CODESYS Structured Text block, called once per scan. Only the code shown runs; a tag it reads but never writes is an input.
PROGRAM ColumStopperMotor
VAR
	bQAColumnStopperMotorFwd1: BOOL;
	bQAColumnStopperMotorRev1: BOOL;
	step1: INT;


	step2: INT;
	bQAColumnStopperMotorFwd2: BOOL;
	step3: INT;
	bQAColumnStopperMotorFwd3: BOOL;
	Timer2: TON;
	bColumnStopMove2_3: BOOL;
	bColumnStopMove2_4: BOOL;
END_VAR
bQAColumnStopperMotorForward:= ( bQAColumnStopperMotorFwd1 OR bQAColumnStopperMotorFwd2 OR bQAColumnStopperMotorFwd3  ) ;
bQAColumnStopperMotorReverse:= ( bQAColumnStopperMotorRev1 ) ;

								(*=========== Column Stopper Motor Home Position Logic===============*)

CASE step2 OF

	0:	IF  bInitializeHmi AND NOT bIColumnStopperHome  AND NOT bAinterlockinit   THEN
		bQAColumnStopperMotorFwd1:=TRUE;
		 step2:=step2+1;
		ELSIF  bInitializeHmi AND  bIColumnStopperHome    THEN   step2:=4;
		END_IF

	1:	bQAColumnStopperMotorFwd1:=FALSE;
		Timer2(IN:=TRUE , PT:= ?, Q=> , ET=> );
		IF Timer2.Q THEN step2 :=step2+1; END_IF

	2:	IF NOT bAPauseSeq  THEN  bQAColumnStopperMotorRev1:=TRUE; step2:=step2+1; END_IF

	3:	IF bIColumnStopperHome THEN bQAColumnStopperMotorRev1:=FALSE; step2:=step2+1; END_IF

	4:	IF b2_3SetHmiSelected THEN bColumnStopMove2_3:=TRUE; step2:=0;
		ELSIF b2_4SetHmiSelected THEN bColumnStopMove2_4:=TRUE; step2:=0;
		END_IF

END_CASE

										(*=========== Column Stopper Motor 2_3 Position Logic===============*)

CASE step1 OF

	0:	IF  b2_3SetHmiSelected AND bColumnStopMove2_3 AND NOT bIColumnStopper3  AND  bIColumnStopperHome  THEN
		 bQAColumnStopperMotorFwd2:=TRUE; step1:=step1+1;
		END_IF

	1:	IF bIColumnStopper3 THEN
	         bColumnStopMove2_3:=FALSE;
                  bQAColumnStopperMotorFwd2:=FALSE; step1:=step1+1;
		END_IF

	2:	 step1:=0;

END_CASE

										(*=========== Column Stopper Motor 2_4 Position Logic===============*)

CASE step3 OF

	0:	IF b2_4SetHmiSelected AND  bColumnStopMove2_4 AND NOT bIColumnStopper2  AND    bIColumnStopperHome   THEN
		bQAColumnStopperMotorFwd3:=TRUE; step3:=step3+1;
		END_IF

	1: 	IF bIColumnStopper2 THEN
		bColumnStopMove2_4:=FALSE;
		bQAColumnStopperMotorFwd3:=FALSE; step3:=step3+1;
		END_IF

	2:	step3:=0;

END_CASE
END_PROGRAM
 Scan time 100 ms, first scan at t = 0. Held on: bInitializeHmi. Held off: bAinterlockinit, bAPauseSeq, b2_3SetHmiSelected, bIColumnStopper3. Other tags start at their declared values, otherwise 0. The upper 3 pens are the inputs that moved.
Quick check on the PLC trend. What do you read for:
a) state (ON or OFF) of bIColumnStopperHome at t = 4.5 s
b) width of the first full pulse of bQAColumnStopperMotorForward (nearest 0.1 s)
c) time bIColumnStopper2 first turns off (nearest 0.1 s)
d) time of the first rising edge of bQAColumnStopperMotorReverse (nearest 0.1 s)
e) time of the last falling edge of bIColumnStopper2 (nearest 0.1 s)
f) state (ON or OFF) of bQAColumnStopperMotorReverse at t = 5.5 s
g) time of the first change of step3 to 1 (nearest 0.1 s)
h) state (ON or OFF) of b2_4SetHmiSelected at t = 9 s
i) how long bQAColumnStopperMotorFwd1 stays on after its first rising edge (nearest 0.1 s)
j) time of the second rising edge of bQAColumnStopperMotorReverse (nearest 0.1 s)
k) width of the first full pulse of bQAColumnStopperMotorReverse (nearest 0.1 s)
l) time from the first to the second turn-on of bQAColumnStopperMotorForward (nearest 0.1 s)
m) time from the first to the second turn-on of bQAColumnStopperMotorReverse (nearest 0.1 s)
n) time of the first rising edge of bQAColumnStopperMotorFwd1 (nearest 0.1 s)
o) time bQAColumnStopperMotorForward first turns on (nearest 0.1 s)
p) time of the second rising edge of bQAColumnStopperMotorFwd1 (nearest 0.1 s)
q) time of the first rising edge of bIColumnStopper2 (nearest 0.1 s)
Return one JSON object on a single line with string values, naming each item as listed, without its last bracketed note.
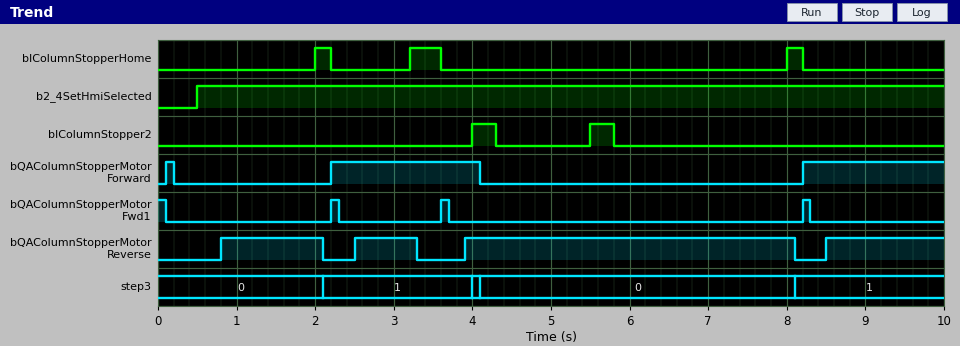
{"state (ON or OFF) of bIColumnStopperHome at t = 4.5 s": "OFF", "width of the first full pulse of bQAColumnStopperMotorForward": "0.1 s", "time bIColumnStopper2 first turns off": "4.3 s", "time of the first rising edge of bQAColumnStopperMotorReverse": "0.8 s", "time of the last falling edge of bIColumnStopper2": "5.8 s", "state (ON or OFF) of bQAColumnStopperMotorReverse at t = 5.5 s": "ON", "time of the first change of step3 to 1": "2.1 s", "state (ON or OFF) of b2_4SetHmiSelected at t = 9 s": "ON", "how long bQAColumnStopperMotorFwd1 stays on after its first rising edge": "0.1 s", "time of the second rising edge of bQAColumnStopperMotorReverse": "2.5 s", "width of the first full pulse of bQAColumnStopperMotorReverse": "1.3 s", "time from the first to the second turn-on of bQAColumnStopperMotorForward": "2.1 s", "time from the first to the second turn-on of bQAColumnStopperMotorReverse": "1.7 s", "time of the first rising edge of bQAColumnStopperMotorFwd1": "2.2 s", "time bQAColumnStopperMotorForward first turns on": "0.1 s", "time of the second rising edge of bQAColumnStopperMotorFwd1": "3.6 s", "time of the first rising edge of bIColumnStopper2": "4.0 s"}
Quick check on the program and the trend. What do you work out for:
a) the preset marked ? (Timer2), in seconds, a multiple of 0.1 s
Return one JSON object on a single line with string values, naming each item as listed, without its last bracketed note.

{"the preset marked ? (Timer2), in seconds, a multiple of 0.1 s": "0.5 s"}
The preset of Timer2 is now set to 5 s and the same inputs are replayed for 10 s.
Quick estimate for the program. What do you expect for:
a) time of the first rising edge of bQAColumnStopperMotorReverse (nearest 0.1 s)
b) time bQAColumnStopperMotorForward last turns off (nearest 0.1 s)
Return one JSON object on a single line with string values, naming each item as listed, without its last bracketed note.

{"time of the first rising edge of bQAColumnStopperMotorReverse": "5.3 s", "time bQAColumnStopperMotorForward last turns off": "0.2 s"}
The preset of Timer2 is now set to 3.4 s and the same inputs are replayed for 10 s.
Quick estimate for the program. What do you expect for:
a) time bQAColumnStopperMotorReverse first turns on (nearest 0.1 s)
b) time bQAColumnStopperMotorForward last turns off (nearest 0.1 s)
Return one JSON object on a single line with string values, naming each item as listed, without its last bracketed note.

{"time bQAColumnStopperMotorReverse first turns on": "3.7 s", "time bQAColumnStopperMotorForward last turns off": "0.2 s"}
